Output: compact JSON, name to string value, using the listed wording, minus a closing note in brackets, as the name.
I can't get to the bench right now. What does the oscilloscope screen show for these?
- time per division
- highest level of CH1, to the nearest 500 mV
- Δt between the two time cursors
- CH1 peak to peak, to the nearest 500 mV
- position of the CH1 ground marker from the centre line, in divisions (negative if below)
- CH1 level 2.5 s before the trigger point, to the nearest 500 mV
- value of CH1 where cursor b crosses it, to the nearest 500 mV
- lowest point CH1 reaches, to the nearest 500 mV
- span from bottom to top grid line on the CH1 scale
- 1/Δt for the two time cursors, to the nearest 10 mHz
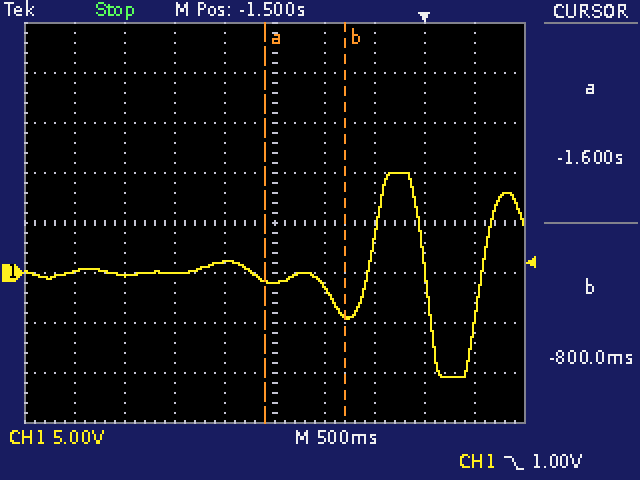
{"time per division": "500 ms", "highest level of CH1, to the nearest 500 mV": "10.0 V", "Δt between the two time cursors": "800 ms", "CH1 peak to peak, to the nearest 500 mV": "20.5 V", "position of the CH1 ground marker from the centre line, in divisions": "-1.0 div", "CH1 level 2.5 s before the trigger point, to the nearest 500 mV": "0.0 V", "value of CH1 where cursor b crosses it, to the nearest 500 mV": "-4.0 V", "lowest point CH1 reaches, to the nearest 500 mV": "-10.5 V", "span from bottom to top grid line on the CH1 scale": "40 V", "1/Δt for the two time cursors, to the nearest 10 mHz": "1.25 Hz"}
